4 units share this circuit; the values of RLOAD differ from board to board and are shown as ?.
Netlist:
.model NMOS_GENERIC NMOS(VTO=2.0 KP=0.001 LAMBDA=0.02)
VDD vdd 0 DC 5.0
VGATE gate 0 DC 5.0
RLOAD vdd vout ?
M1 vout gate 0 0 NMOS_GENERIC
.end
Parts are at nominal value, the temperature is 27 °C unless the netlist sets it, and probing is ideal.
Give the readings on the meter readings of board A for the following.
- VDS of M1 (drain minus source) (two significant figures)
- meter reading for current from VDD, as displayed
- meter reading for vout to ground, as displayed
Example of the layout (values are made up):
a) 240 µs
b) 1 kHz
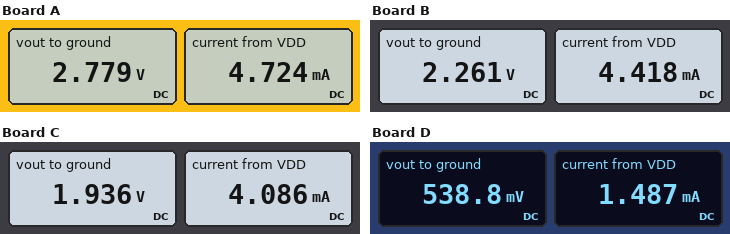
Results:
a) 2.8 V
b) 4.724 mA
c) 2.779 V
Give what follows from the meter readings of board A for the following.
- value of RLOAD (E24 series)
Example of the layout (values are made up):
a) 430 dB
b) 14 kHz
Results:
a) 470 Ω
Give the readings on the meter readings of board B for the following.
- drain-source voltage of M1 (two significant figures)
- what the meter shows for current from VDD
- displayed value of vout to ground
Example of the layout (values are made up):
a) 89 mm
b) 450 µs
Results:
a) 2.3 V
b) 4.418 mA
c) 2.261 V
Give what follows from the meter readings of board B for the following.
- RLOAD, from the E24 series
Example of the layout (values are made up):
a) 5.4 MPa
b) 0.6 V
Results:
a) 620 Ω
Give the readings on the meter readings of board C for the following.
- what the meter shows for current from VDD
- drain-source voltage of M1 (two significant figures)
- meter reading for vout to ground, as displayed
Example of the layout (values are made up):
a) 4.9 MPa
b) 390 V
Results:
a) 4.086 mA
b) 1.9 V
c) 1.936 V
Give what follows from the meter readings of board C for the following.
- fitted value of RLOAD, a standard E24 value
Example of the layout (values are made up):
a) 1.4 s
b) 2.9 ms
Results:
a) 750 Ω
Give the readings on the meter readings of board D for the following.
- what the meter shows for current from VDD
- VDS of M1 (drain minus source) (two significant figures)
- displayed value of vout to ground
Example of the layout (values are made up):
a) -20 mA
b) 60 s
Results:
a) 1.487 mA
b) 540 mV
c) 538.8 mV
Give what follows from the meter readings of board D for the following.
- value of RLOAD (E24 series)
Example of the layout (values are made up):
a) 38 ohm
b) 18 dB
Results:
a) 3 kΩ
